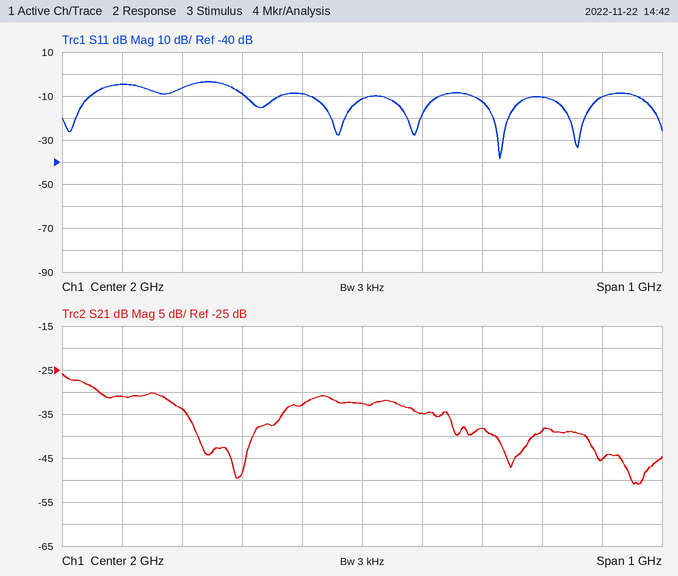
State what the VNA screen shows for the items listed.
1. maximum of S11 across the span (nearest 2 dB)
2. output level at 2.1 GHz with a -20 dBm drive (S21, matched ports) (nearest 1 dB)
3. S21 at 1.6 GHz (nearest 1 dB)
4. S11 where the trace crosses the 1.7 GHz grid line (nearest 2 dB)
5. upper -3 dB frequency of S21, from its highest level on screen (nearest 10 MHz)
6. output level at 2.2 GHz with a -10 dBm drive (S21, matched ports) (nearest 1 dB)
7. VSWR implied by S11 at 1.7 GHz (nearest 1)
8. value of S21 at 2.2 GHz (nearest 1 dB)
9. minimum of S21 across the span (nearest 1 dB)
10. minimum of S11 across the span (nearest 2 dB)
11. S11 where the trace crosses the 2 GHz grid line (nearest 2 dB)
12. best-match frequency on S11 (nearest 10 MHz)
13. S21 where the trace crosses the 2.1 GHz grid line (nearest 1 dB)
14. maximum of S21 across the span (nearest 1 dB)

-4 dB
-55 dBm
-31 dB
-6 dB
1.55 GHz
-48 dBm
3
-38 dB
-51 dB
-38 dB
-12 dB
2.23 GHz
-35 dB
-26 dB
